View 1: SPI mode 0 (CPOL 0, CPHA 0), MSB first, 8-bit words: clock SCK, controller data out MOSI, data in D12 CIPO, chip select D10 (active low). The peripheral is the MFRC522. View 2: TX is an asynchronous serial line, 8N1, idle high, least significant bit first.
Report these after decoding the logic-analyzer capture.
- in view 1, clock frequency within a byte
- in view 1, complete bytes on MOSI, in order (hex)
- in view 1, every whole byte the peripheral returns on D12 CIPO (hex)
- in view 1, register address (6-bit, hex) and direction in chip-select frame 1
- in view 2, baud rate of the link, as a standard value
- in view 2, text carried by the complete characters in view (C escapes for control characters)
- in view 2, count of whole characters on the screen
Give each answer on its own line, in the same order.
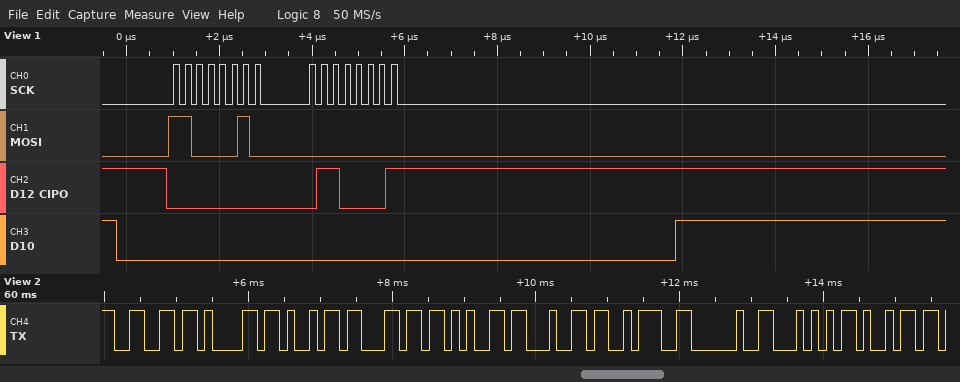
4 MHz
0xC2 0x00
0x00 0x61
0x21 read
9600 baud
"failed: Ti"
10
